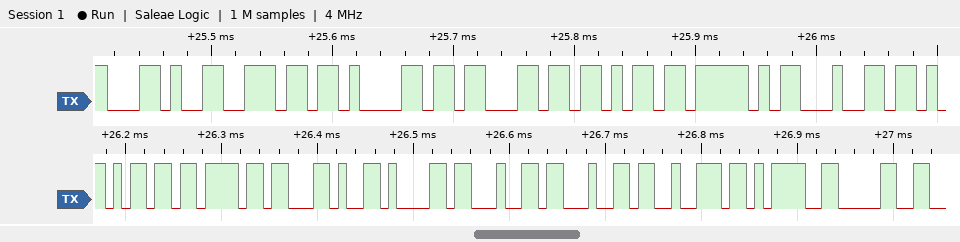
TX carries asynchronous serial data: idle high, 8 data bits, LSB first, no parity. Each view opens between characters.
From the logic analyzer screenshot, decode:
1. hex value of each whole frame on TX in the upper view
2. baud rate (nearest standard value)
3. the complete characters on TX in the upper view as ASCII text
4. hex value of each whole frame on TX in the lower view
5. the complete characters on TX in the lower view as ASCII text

2C, 6E, 61, 63, 6B, 5F, 64
115200 baud
",nack_d"
6D, 6F, 2C, 61, 64, 64, 72, 3D, 30
"mo,addr=0"
